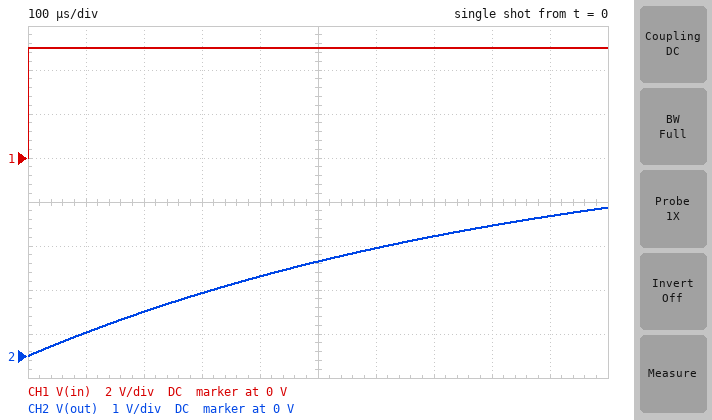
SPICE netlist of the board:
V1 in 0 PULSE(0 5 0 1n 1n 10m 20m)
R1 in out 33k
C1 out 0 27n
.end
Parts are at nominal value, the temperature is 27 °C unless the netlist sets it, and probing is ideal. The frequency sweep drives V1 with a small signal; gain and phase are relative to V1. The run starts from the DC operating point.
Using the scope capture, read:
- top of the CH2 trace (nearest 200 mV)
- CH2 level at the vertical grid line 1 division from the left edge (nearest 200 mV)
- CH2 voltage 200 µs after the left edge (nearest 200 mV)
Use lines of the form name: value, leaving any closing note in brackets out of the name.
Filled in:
top of the CH2 trace: 3.4 V
CH2 level at the vertical grid line 1 division from the left edge: 600 mV
CH2 voltage 200 µs after the left edge: 1.0 V
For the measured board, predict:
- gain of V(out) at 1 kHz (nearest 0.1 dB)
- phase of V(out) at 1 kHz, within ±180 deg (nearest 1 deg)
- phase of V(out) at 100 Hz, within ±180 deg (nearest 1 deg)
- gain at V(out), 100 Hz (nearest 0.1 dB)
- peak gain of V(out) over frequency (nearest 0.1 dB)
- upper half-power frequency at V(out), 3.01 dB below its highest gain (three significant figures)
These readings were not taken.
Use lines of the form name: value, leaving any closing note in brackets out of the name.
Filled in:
gain of V(out) at 1 kHz: -15.1 dB
phase of V(out) at 1 kHz, within ±180 deg: -80 deg
phase of V(out) at 100 Hz, within ±180 deg: -29 deg
gain at V(out), 100 Hz: -1.2 dB
peak gain of V(out) over frequency: 0 dB
upper half-power frequency at V(out), 3.01 dB below its highest gain: 179 Hz
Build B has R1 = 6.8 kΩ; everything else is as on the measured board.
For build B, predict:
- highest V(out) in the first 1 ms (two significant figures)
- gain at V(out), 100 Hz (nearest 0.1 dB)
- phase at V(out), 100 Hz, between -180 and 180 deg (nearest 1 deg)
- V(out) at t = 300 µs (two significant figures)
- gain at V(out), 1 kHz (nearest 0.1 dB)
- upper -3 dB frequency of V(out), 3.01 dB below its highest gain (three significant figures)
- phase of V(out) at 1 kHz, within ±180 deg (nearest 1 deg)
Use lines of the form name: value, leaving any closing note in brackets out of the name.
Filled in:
highest V(out) in the first 1 ms: 5.0 V
gain at V(out), 100 Hz: -0.1 dB
phase at V(out), 100 Hz, between -180 and 180 deg: -7 deg
V(out) at t = 300 µs: 4.0 V
gain at V(out), 1 kHz: -3.7 dB
upper -3 dB frequency of V(out), 3.01 dB below its highest gain: 867 Hz
phase of V(out) at 1 kHz, within ±180 deg: -49 deg
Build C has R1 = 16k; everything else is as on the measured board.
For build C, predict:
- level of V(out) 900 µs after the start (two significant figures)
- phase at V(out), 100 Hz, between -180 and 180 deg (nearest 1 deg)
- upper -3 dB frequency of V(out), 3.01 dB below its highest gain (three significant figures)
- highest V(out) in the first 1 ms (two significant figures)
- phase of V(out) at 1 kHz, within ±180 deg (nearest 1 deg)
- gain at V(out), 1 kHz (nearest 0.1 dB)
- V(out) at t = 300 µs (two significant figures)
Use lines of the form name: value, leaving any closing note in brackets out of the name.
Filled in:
level of V(out) 900 µs after the start: 4.4 V
phase at V(out), 100 Hz, between -180 and 180 deg: -15 deg
upper -3 dB frequency of V(out), 3.01 dB below its highest gain: 368 Hz
highest V(out) in the first 1 ms: 4.5 V
phase of V(out) at 1 kHz, within ±180 deg: -70 deg
gain at V(out), 1 kHz: -9.2 dB
V(out) at t = 300 µs: 2.5 V
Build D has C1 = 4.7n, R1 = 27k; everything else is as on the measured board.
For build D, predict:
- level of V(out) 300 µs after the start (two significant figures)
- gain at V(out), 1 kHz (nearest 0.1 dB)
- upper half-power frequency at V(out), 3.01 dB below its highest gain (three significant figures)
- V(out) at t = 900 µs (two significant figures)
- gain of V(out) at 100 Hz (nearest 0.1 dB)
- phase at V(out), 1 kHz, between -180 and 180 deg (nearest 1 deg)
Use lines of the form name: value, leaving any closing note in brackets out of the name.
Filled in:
level of V(out) 300 µs after the start: 4.5 V
gain at V(out), 1 kHz: -2.1 dB
upper half-power frequency at V(out), 3.01 dB below its highest gain: 1.25 kHz
V(out) at t = 900 µs: 5.0 V
gain of V(out) at 100 Hz: 0 dB
phase at V(out), 1 kHz, between -180 and 180 deg: -39 deg
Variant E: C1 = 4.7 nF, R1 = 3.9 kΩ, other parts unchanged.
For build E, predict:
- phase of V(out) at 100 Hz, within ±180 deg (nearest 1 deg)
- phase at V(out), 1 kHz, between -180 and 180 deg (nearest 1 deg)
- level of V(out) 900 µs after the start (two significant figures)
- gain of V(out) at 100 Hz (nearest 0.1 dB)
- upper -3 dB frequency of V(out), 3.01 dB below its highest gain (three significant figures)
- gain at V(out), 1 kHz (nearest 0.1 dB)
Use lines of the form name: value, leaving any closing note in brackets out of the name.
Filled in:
phase of V(out) at 100 Hz, within ±180 deg: -1 deg
phase at V(out), 1 kHz, between -180 and 180 deg: -7 deg
level of V(out) 900 µs after the start: 5.0 V
gain of V(out) at 100 Hz: 0 dB
upper -3 dB frequency of V(out), 3.01 dB below its highest gain: 8.68 kHz
gain at V(out), 1 kHz: -0.1 dB
